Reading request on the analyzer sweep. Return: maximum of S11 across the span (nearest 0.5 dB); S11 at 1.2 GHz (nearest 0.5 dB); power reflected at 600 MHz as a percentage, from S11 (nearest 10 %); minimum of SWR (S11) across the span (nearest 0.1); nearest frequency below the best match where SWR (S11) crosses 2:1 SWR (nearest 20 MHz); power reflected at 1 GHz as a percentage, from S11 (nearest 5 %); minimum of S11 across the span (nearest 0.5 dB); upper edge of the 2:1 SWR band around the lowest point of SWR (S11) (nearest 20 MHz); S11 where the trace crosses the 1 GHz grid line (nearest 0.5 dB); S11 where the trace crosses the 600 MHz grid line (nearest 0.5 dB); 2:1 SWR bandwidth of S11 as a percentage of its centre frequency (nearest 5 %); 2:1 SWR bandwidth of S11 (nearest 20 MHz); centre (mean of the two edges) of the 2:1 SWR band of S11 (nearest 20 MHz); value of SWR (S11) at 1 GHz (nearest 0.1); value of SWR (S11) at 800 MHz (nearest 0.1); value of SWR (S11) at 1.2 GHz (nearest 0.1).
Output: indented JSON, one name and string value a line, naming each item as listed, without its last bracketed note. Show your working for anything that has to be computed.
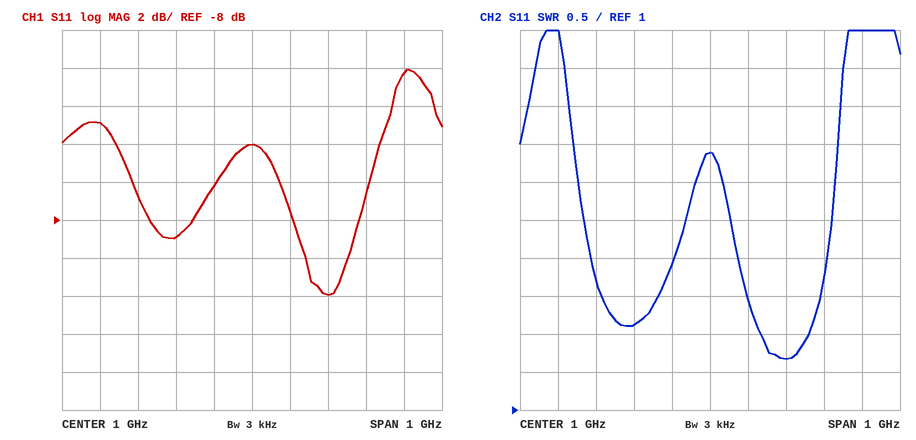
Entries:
{
  "maximum of S11 across the span": "0.0 dB",
  "S11 at 1.2 GHz": "-12.0 dB",
  "power reflected at 600 MHz as a percentage, from S11": "10^(-3/10) ≈ 50 %",
  "minimum of SWR (S11) across the span": "1.7",
  "nearest frequency below the best match where SWR (S11) crosses 2:1 SWR": "1.14 GHz",
  "power reflected at 1 GHz as a percentage, from S11": "10^(-4/10) ≈ 40 %",
  "minimum of S11 across the span": "-12.0 dB",
  "upper edge of the 2:1 SWR band around the lowest point of SWR (S11)": "1.26 GHz",
  "S11 where the trace crosses the 1 GHz grid line": "-4.0 dB",
  "S11 where the trace crosses the 600 MHz grid line": "-3.0 dB",
  "2:1 SWR bandwidth of S11 as a percentage of its centre frequency": "120 MHz / 1.2 GHz ≈ 10 %",
  "2:1 SWR bandwidth of S11": "1.26 GHz − 1.14 GHz = 120 MHz",
  "centre (mean of the two edges) of the 2:1 SWR band of S11": "1.20 GHz",
  "value of SWR (S11) at 1 GHz": "4.4",
  "value of SWR (S11) at 800 MHz": "2.1",
  "value of SWR (S11) at 1.2 GHz": "1.7"
}
